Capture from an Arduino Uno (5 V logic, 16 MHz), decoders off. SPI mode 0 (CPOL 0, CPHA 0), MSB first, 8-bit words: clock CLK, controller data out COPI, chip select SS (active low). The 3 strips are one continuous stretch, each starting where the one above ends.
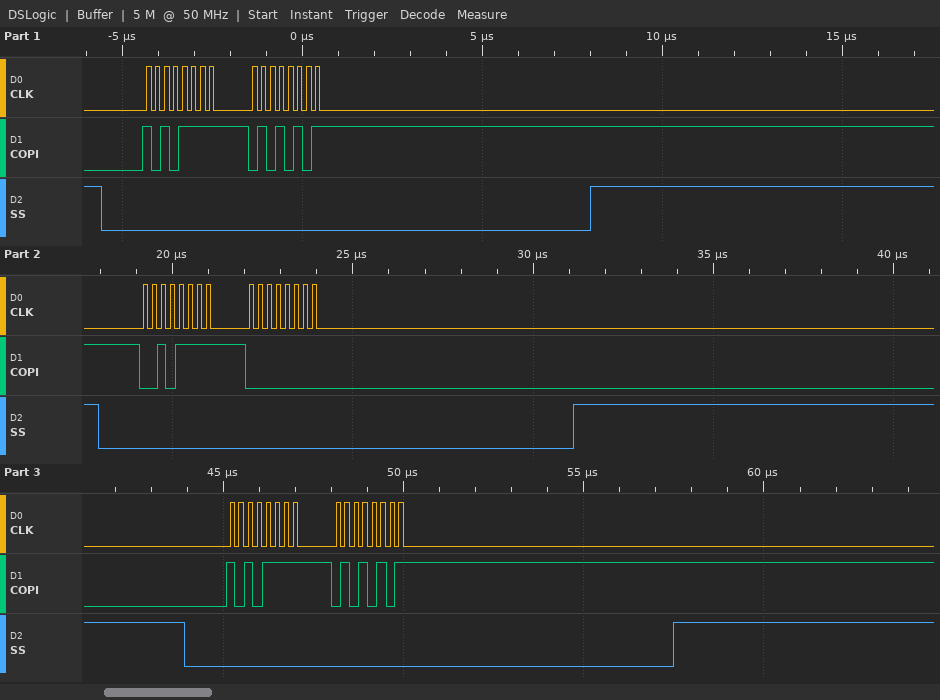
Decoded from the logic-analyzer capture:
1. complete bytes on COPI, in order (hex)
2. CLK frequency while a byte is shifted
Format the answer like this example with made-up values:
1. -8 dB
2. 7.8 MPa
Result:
1. 0xAF 0x55 0x2F 0x00 0xAF 0x55
2. 4 MHz
